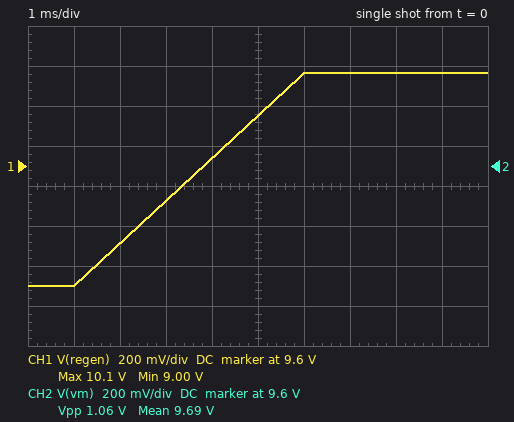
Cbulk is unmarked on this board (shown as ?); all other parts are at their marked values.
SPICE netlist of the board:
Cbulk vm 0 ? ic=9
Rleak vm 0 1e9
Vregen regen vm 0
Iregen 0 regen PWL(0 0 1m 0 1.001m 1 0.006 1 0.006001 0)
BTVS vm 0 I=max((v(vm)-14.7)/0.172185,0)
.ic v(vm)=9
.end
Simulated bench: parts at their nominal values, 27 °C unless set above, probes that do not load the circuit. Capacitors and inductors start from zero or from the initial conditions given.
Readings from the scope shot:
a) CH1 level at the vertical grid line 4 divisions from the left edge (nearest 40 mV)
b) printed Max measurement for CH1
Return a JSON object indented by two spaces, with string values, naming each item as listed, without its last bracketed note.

{
  "CH1 level at the vertical grid line 4 divisions from the left edge": "9.64 V",
  "printed Max measurement for CH1": "10.1 V"
}
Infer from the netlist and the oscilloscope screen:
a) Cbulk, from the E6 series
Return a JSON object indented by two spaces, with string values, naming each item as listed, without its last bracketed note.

{
  "Cbulk, from the E6 series": "4.7 mF"
}
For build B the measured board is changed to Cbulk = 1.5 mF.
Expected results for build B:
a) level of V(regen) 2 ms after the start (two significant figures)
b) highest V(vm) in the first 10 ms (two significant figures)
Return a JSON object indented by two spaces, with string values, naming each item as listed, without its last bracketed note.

{
  "level of V(regen) 2 ms after the start": "9.7 V",
  "highest V(vm) in the first 10 ms": "12 V"
}
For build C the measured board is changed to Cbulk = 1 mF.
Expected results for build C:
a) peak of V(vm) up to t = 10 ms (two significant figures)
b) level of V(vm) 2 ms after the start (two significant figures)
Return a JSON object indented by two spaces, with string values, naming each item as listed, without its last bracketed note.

{
  "peak of V(vm) up to t = 10 ms": "14 V",
  "level of V(vm) 2 ms after the start": "10 V"
}
